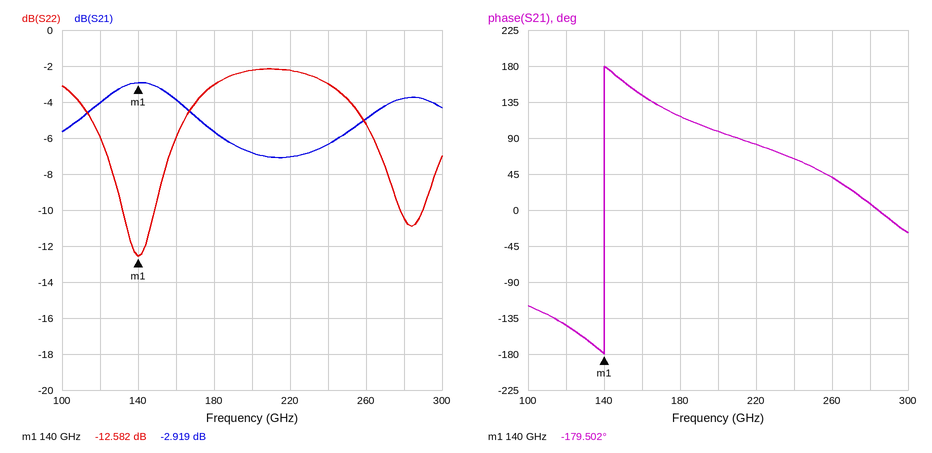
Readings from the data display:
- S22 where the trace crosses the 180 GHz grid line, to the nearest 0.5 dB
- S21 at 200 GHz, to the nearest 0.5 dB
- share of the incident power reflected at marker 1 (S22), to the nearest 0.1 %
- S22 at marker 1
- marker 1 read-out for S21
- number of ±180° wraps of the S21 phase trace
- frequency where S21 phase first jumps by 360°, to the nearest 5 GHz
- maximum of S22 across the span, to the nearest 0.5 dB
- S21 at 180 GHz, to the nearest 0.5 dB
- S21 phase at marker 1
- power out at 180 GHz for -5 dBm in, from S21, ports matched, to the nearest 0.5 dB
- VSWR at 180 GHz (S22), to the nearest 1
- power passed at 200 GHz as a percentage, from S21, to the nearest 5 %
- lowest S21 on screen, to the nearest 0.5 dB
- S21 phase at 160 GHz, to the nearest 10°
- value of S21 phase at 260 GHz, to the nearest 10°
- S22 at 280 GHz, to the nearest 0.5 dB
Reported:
-3.0 dB
-7.0 dB
5.5 %
-12.582 dB
-2.919 dB
1
140 GHz
-2.0 dB
-5.5 dB
-179.502°
-10.5 dBm
6
20 %
-7.0 dB
140°
40°
-10.5 dB
